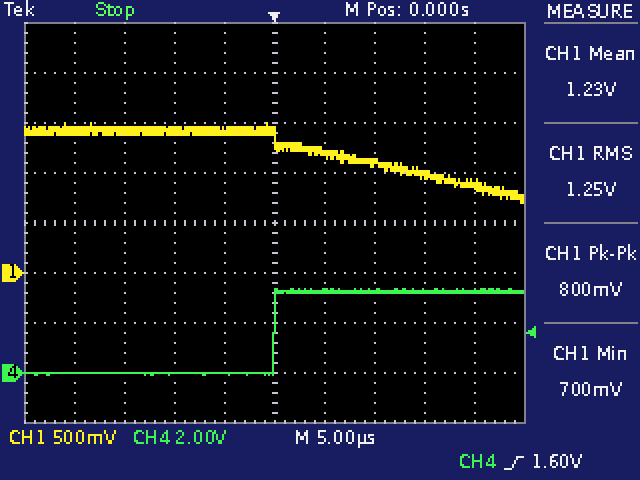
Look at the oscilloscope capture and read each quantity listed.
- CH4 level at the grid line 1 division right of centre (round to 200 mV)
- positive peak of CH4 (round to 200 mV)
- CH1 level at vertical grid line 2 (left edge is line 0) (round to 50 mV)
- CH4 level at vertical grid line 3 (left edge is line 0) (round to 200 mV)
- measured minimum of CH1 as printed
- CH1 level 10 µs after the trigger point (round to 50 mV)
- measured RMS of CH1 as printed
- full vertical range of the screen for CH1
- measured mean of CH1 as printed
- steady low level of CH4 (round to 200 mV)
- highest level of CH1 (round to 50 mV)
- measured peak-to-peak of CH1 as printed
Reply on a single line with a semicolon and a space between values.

3.2 V; 3.4 V; 1.40 V; 0.0 V; 700 mV; 1.10 V; 1.25 V; 4 V; 1.23 V; 0.0 V; 1.50 V; 800 mV
